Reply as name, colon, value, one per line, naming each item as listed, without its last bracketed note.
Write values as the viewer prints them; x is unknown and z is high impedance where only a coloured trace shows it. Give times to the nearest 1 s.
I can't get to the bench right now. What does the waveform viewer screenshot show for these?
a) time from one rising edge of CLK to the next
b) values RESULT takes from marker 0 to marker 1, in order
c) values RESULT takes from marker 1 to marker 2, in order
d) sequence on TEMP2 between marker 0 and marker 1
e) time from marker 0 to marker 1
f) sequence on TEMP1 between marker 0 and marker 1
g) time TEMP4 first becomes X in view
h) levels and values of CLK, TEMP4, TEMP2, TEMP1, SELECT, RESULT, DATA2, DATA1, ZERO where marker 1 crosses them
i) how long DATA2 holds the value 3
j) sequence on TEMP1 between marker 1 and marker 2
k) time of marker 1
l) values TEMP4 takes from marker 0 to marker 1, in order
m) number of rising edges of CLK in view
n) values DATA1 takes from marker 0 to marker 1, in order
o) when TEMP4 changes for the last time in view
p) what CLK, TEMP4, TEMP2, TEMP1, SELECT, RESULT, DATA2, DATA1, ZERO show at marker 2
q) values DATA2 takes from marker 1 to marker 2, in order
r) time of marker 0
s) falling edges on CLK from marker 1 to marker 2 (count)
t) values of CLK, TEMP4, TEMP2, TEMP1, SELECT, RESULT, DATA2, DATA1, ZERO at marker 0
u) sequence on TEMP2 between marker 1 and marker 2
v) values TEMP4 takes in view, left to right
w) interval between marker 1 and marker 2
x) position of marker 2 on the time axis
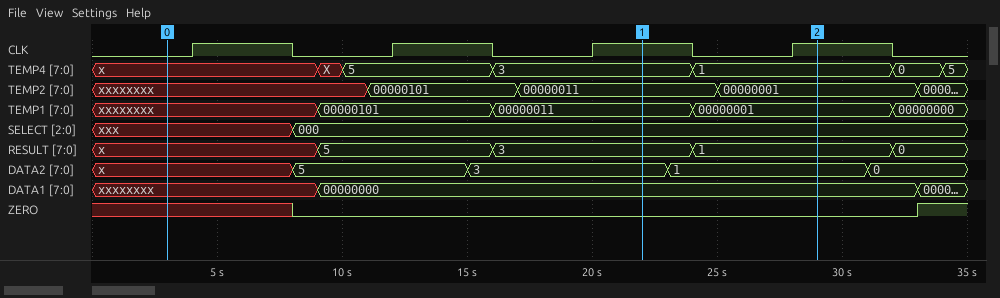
time from one rising edge of CLK to the next: 8 s
values RESULT takes from marker 0 to marker 1, in order: x, 5, 3
values RESULT takes from marker 1 to marker 2, in order: 3, 1
sequence on TEMP2 between marker 0 and marker 1: xxxxxxxx, 00000101, 00000011
time from marker 0 to marker 1: 19 s
sequence on TEMP1 between marker 0 and marker 1: xxxxxxxx, 00000101, 00000011
time TEMP4 first becomes X in view: 9 s
levels and values of CLK, TEMP4, TEMP2, TEMP1, SELECT, RESULT, DATA2, DATA1, ZERO where marker 1 crosses them: CLK=1, TEMP4=3, TEMP2=00000011, TEMP1=00000011, SELECT=000, RESULT=3, DATA2=3, DATA1=00000000, ZERO=0
how long DATA2 holds the value 3: 8 s
sequence on TEMP1 between marker 1 and marker 2: 00000011, 00000001
time of marker 1: 22 s
values TEMP4 takes from marker 0 to marker 1, in order: x, X, 5, 3
number of rising edges of CLK in view: 4
values DATA1 takes from marker 0 to marker 1, in order: xxxxxxxx, 00000000
when TEMP4 changes for the last time in view: 34 s
what CLK, TEMP4, TEMP2, TEMP1, SELECT, RESULT, DATA2, DATA1, ZERO show at marker 2: CLK=1, TEMP4=1, TEMP2=00000001, TEMP1=00000001, SELECT=000, RESULT=1, DATA2=1, DATA1=00000000, ZERO=0
values DATA2 takes from marker 1 to marker 2, in order: 3, 1
time of marker 0: 3 s
falling edges on CLK from marker 1 to marker 2: 1
values of CLK, TEMP4, TEMP2, TEMP1, SELECT, RESULT, DATA2, DATA1, ZERO at marker 0: CLK=0, TEMP4=x, TEMP2=xxxxxxxx, TEMP1=xxxxxxxx, SELECT=xxx, RESULT=x, DATA2=x, DATA1=xxxxxxxx, ZERO=x
sequence on TEMP2 between marker 1 and marker 2: 00000011, 00000001
values TEMP4 takes in view, left to right: x, X, 5, 3, 1, 0, 5
interval between marker 1 and marker 2: 7 s
position of marker 2 on the time axis: 29 s
